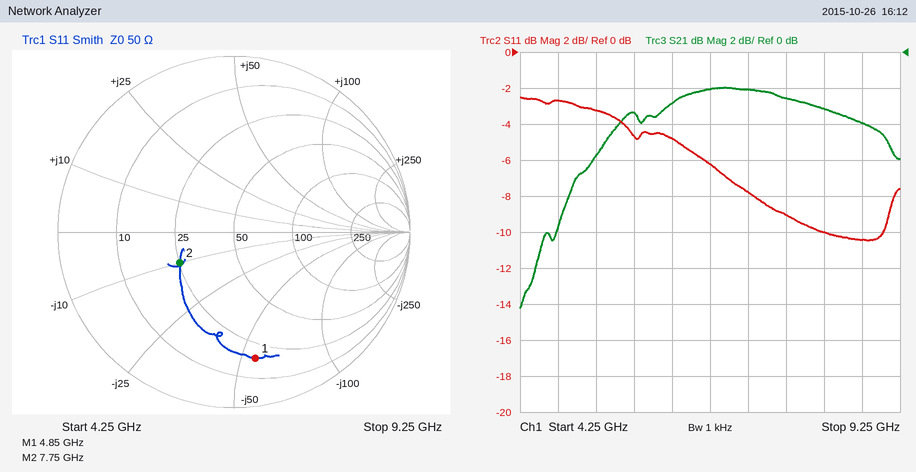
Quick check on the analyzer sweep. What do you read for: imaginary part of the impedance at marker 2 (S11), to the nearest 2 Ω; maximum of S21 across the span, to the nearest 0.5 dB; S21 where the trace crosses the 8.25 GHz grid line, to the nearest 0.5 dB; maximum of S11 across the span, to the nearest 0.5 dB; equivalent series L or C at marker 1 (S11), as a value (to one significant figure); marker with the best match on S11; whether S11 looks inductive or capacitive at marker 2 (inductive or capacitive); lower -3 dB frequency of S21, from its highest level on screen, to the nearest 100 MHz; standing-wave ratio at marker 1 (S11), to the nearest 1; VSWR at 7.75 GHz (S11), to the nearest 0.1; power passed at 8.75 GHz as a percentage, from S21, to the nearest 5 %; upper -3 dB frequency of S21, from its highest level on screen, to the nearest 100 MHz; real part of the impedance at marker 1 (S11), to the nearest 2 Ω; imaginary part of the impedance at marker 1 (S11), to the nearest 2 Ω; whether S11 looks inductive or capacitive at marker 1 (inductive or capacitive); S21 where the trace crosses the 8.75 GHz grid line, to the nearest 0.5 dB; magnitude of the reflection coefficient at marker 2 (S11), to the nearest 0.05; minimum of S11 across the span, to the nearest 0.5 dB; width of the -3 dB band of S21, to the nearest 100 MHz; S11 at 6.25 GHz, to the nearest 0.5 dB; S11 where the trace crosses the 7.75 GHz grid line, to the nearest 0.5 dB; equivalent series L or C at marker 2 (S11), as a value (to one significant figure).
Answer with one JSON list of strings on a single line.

["-10 Ω", "-2.0 dB", "-3.0 dB", "-2.5 dB", "600 fF", "marker 2", "capacitive", "5.4 GHz", "6", "2.1", "40 %", "9.1 GHz", "18 Ω", "-56 Ω", "capacitive", "-4.0 dB", "0.35", "-10.5 dB", "3.7 GHz", "-5.0 dB", "-9.0 dB", "2 pF"]
